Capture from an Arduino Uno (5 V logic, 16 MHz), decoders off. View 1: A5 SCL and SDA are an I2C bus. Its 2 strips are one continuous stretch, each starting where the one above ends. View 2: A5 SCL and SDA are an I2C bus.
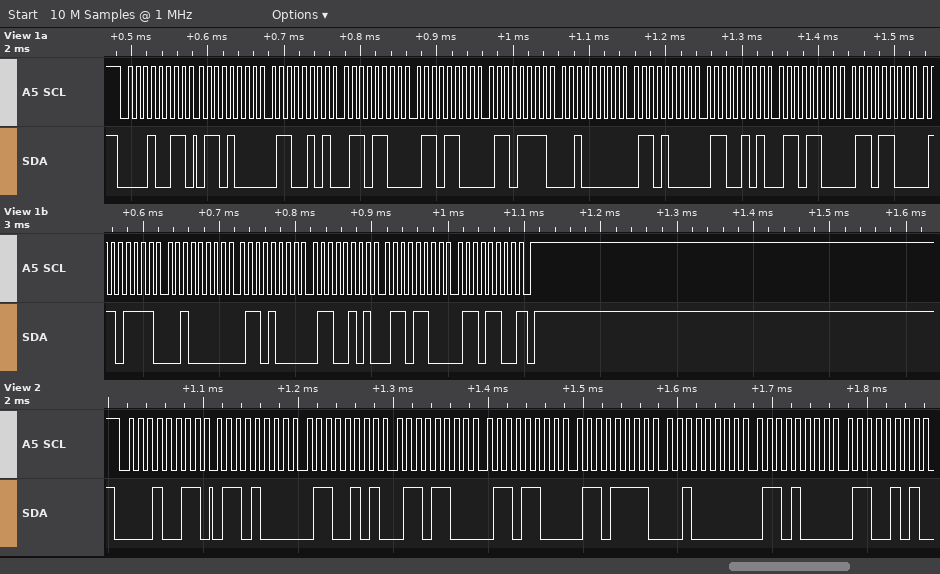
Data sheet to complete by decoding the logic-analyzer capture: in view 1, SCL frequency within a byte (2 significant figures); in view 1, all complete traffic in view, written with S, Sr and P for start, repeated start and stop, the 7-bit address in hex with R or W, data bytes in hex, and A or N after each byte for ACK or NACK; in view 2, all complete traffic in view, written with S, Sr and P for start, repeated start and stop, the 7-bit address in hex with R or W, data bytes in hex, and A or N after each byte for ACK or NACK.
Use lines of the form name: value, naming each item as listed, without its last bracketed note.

in view 1, SCL frequency within a byte: 100 kHz
in view 1, all complete traffic in view, written with S, Sr and P for start, repeated start and stop, the 7-bit address in hex with R or W, data bytes in hex, and A or N after each byte for ACK or NACK: S 09R A 68 A 65 A 6C A 6C A 6F A 20 A 68 A 65 A 6C A 6C A 6F A 20 A 68 A 65 A 6C A 6C N P
in view 2, all complete traffic in view, written with S, Sr and P for start, repeated start and stop, the 7-bit address in hex with R or W, data bytes in hex, and A or N after each byte for ACK or NACK: S 09R A 68 A 65 A 6C A 6C A 6F A 20 A 68 A 65 A
